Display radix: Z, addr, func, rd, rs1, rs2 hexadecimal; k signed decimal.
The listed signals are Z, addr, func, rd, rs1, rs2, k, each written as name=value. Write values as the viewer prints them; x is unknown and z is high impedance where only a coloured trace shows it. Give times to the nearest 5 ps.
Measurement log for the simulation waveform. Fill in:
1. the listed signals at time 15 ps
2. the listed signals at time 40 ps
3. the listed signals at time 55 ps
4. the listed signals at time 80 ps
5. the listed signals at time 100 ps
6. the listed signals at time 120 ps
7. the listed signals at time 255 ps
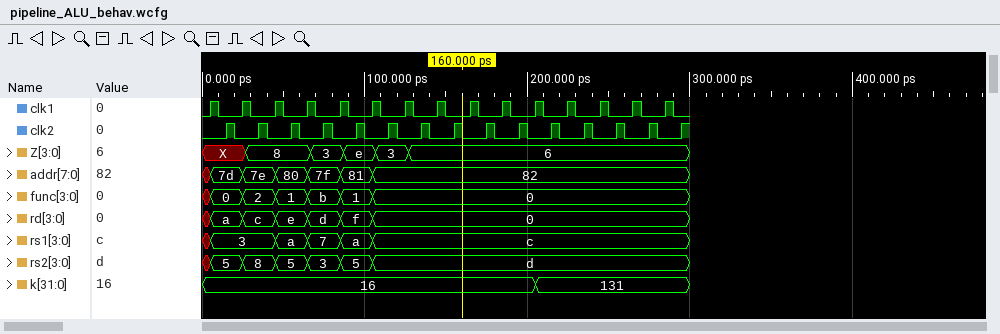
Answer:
Z=X, addr=7d, func=0, rd=a, rs1=3, rs2=5, k=16
Z=8, addr=7e, func=2, rd=c, rs1=3, rs2=8, k=16
Z=8, addr=80, func=1, rd=e, rs1=a, rs2=5, k=16
Z=3, addr=7f, func=b, rd=d, rs1=7, rs2=3, k=16
Z=e, addr=81, func=1, rd=f, rs1=a, rs2=5, k=16
Z=3, addr=82, func=0, rd=0, rs1=c, rs2=d, k=16
Z=6, addr=82, func=0, rd=0, rs1=c, rs2=d, k=131
